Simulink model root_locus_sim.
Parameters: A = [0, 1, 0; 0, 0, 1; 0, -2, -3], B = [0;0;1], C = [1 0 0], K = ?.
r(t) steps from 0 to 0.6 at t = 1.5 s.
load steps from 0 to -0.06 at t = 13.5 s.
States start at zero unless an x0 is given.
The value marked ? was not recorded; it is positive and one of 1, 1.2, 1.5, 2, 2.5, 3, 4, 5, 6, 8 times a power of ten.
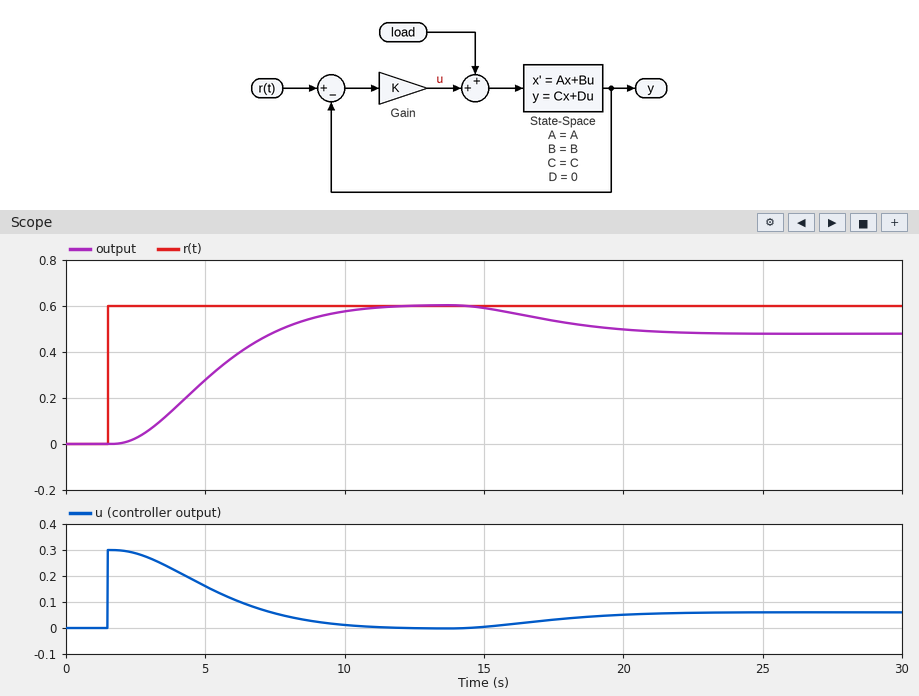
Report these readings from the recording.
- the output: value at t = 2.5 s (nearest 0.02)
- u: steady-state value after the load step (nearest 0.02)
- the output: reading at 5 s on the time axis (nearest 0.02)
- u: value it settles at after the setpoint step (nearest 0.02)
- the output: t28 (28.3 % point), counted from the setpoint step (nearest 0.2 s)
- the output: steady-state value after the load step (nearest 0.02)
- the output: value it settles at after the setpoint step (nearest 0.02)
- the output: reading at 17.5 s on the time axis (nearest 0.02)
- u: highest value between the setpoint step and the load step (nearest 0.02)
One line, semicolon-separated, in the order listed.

0.02; 0.06; 0.28; 0.00; 2.6 s; 0.48; 0.60; 0.54; 0.30
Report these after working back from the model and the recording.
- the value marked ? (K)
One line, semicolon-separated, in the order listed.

0.5
